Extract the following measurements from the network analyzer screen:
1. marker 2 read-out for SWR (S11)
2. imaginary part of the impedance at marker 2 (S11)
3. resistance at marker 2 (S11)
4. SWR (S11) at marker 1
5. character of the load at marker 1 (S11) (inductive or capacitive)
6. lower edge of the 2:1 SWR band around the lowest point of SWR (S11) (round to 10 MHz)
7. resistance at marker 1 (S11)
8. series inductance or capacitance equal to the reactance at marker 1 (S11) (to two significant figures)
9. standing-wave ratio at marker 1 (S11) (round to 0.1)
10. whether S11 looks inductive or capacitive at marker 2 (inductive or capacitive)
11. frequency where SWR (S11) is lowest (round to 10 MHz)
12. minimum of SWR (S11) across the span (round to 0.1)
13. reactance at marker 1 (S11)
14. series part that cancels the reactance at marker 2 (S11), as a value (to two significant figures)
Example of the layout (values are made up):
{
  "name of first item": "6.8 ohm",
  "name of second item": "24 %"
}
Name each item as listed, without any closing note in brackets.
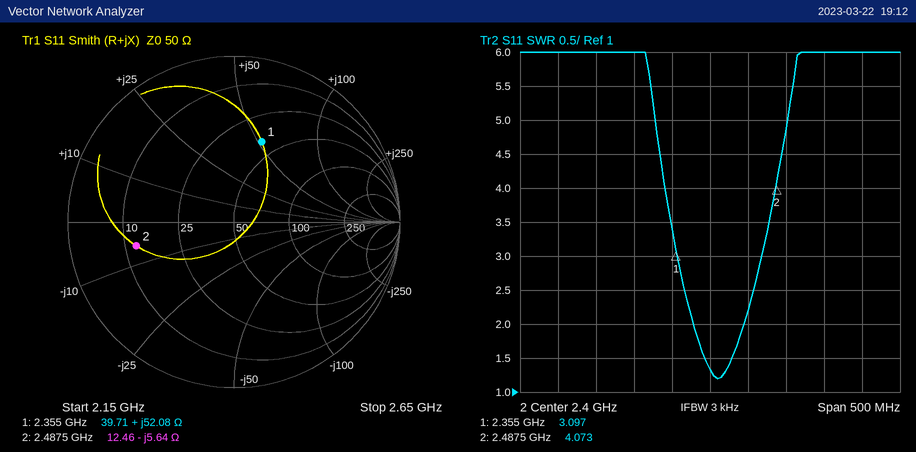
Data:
{
  "marker 2 read-out for SWR": "4.073",
  "imaginary part of the impedance at marker 2": "-5.64 Ω",
  "resistance at marker 2": "12.46 Ω",
  "SWR (S11) at marker 1": "3.097",
  "character of the load at marker 1 (S11)": "inductive",
  "lower edge of the 2:1 SWR band around the lowest point of SWR (S11)": "2.38 GHz",
  "resistance at marker 1": "39.71 Ω",
  "series inductance or capacitance equal to the reactance at marker 1 (S11)": "3.5 nH",
  "standing-wave ratio at marker 1 (S11)": "3.1",
  "whether S11 looks inductive or capacitive at marker 2": "capacitive",
  "frequency where SWR (S11) is lowest": "2.41 GHz",
  "minimum of SWR (S11) across the span": "1.2",
  "reactance at marker 1": "+52.08 Ω",
  "series part that cancels the reactance at marker 2 (S11), as a value": "360 pH"
}
